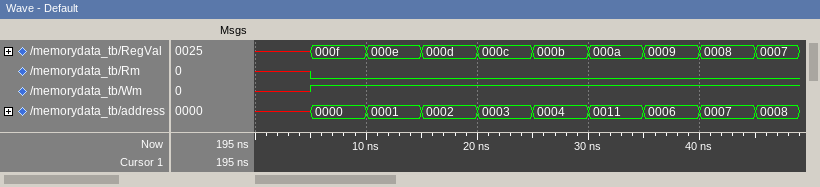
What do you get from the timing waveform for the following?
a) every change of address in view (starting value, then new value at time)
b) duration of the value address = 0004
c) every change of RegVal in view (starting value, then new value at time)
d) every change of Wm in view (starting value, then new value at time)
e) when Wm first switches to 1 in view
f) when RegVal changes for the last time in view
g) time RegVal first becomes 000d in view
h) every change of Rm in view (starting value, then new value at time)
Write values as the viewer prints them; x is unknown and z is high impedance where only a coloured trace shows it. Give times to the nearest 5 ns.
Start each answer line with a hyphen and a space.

- x, 0000 at 5 ns, 0001 at 10 ns, 0002 at 15 ns, 0003 at 20 ns, 0004 at 25 ns, 0011 at 30 ns, 0006 at 35 ns, 0007 at 40 ns, 0008 at 45 ns
- 5 ns
- x, 000f at 5 ns, 000e at 10 ns, 000d at 15 ns, 000c at 20 ns, 000b at 25 ns, 000a at 30 ns, 0009 at 35 ns, 0008 at 40 ns, 0007 at 45 ns
- x, 1 at 5 ns
- 5 ns
- 45 ns
- 15 ns
- x, 0 at 5 ns
